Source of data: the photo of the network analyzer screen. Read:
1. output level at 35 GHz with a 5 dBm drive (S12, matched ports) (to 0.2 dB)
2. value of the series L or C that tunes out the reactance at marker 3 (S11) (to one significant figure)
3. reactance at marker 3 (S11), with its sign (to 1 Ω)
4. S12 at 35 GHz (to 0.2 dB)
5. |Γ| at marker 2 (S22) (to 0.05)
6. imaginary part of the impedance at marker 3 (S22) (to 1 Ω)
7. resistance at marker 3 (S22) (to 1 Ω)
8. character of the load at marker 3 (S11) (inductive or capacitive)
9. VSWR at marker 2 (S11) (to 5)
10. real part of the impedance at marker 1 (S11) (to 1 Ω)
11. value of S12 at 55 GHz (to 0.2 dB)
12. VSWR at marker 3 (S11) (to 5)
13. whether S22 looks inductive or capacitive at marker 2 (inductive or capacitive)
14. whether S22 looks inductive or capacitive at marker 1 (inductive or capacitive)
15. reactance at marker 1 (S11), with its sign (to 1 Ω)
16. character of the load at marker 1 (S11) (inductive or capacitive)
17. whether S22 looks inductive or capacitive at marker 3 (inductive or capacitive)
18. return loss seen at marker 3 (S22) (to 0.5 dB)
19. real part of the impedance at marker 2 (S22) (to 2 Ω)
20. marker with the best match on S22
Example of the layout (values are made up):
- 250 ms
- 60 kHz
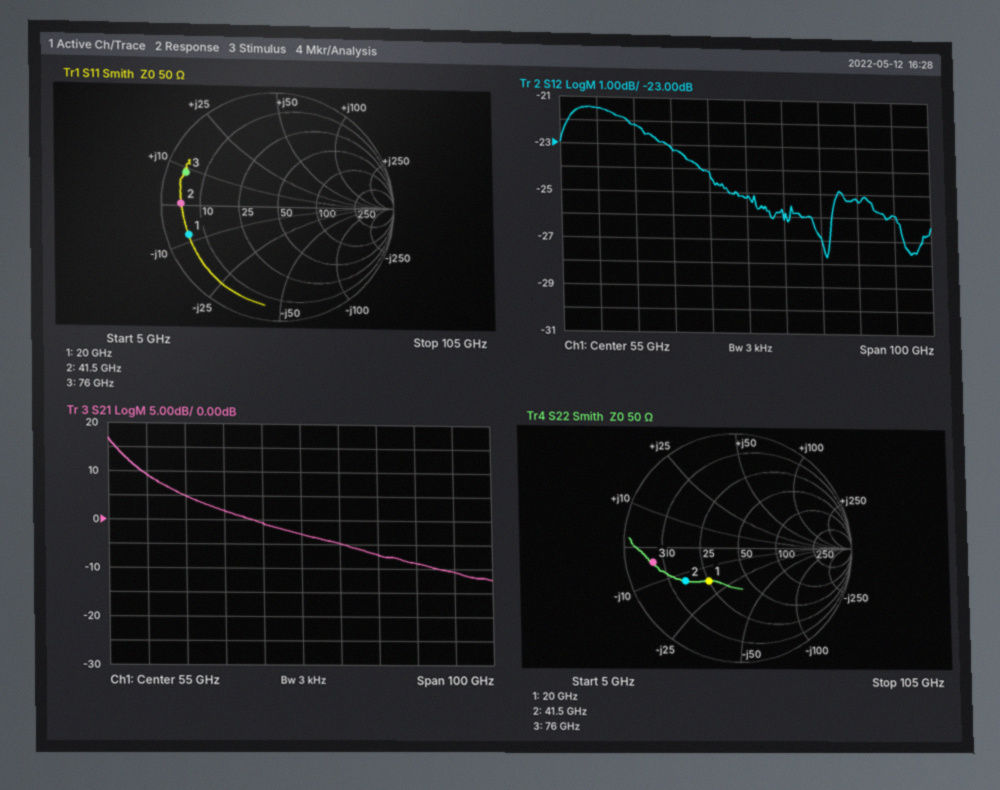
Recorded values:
- -18.2 dBm
- 200 fF
- +9 Ω
- -23.2 dB
- 0.55
- -4 Ω
- 7 Ω
- inductive
- 10
- 5 Ω
- -25.2 dB
- 10
- capacitive
- capacitive
- -8 Ω
- capacitive
- capacitive
- 2.5 dB
- 16 Ω
- marker 1
